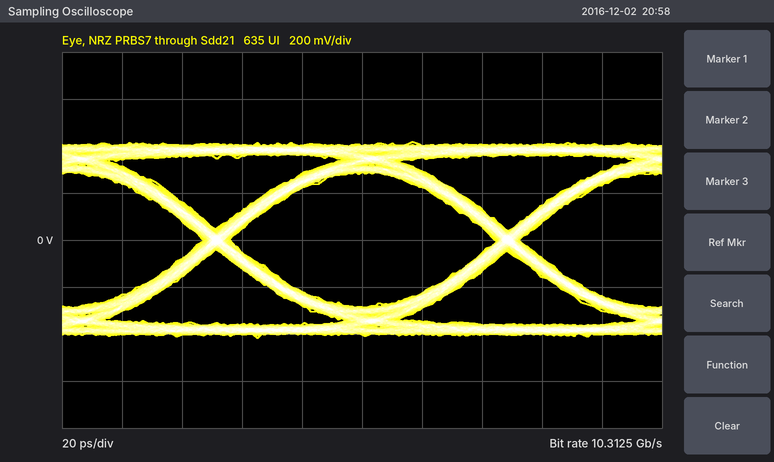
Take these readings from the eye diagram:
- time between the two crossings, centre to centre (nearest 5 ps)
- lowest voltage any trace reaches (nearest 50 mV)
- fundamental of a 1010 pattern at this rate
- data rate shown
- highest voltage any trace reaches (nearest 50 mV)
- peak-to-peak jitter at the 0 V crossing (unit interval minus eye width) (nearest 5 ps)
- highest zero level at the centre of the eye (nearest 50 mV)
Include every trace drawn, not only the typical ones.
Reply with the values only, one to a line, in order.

95 ps
-400 mV
5.15625 GHz
10.3125 Gb/s
400 mV
10 ps
-300 mV
